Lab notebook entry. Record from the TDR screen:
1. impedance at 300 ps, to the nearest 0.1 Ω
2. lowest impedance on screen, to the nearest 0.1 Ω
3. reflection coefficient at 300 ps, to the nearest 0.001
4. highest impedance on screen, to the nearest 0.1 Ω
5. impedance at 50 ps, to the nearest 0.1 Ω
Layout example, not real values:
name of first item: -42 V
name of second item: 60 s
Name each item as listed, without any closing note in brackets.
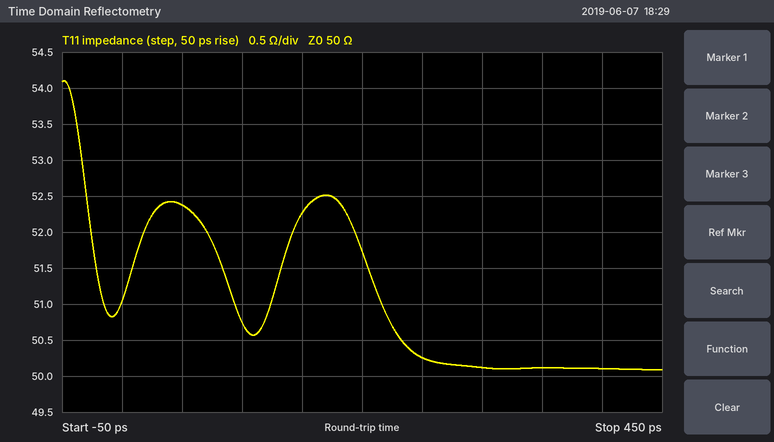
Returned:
impedance at 300 ps, to the nearest 0.1 Ω: 50.1 Ω
lowest impedance on screen, to the nearest 0.1 Ω: 50.1 Ω
reflection coefficient at 300 ps, to the nearest 0.001: +0.001
highest impedance on screen, to the nearest 0.1 Ω: 54.1 Ω
impedance at 50 ps, to the nearest 0.1 Ω: 52.4 Ω
